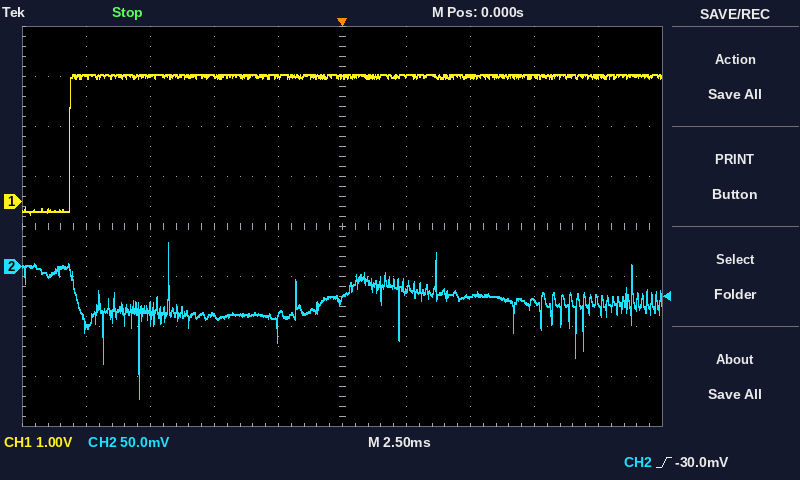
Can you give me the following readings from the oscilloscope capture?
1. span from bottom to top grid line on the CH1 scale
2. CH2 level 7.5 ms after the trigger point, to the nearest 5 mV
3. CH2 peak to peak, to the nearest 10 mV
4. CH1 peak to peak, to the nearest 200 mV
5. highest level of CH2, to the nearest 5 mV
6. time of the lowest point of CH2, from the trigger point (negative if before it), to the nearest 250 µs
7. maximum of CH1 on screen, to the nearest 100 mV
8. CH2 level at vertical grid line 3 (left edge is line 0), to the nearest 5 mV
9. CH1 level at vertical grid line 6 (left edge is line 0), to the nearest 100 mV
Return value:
8 V
-35 mV
160 mV
2.8 V
25 mV
-8.00 ms
2.5 V
-50 mV
2.5 V
